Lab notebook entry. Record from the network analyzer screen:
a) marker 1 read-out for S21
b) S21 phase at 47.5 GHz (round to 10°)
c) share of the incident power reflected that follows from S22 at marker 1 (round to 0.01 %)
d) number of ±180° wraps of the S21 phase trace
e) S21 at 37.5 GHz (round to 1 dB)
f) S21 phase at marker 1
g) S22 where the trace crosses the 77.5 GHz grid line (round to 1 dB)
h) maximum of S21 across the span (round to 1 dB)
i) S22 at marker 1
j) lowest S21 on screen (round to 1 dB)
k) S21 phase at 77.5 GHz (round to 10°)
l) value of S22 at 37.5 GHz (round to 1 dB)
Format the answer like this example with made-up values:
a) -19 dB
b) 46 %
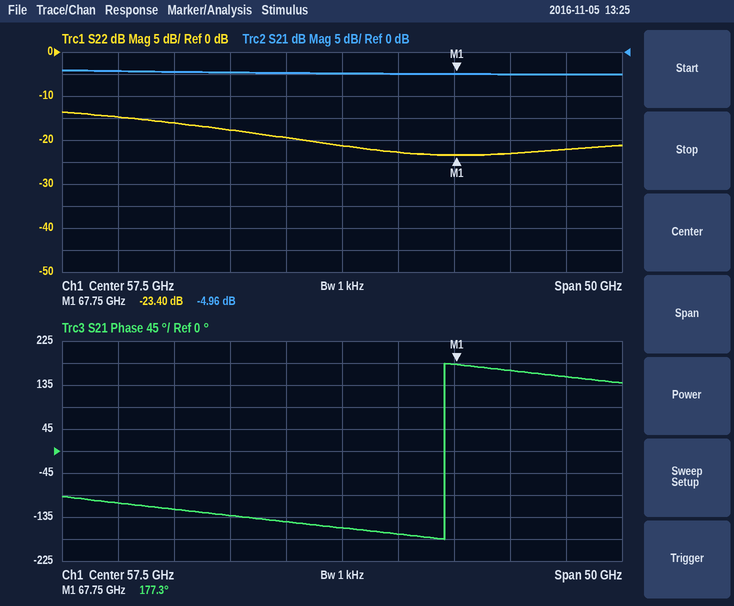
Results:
a) -4.96 dB
b) -130°
c) 0.46 %
d) 1
e) -4 dB
f) 177.3°
g) -22 dB
h) -4 dB
i) -23.40 dB
j) -5 dB
k) 150°
l) -15 dB
